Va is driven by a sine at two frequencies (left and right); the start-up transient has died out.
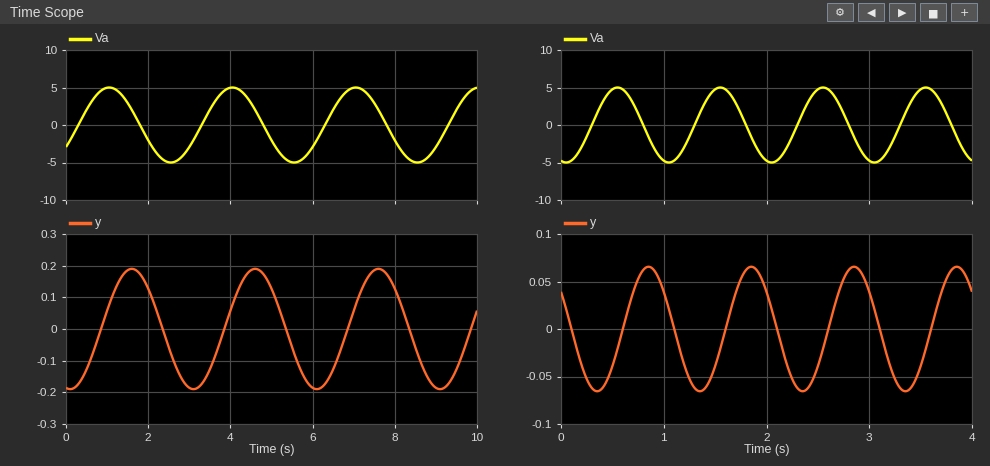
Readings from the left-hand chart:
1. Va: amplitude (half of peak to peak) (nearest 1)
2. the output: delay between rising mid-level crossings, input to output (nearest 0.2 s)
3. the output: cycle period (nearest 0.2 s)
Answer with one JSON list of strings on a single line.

["5", "0.6 s", "3.0 s"]
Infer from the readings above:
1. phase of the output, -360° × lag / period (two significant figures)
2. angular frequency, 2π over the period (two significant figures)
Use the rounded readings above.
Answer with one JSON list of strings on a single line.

["-72°", "2.1 rad/s"]
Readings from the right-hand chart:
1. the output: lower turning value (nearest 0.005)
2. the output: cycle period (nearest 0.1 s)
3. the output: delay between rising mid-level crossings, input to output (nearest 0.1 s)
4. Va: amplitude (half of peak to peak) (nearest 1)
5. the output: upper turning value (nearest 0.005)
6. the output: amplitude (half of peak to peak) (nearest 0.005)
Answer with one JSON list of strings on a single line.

["-0.065", "1.0 s", "0.3 s", "5", "0.065", "0.065"]
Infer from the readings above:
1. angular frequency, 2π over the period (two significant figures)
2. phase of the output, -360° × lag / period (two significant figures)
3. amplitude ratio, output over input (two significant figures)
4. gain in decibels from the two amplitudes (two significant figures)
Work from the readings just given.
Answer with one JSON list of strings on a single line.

["6.3 rad/s", "-110°", "0.013", "-38 dB"]
